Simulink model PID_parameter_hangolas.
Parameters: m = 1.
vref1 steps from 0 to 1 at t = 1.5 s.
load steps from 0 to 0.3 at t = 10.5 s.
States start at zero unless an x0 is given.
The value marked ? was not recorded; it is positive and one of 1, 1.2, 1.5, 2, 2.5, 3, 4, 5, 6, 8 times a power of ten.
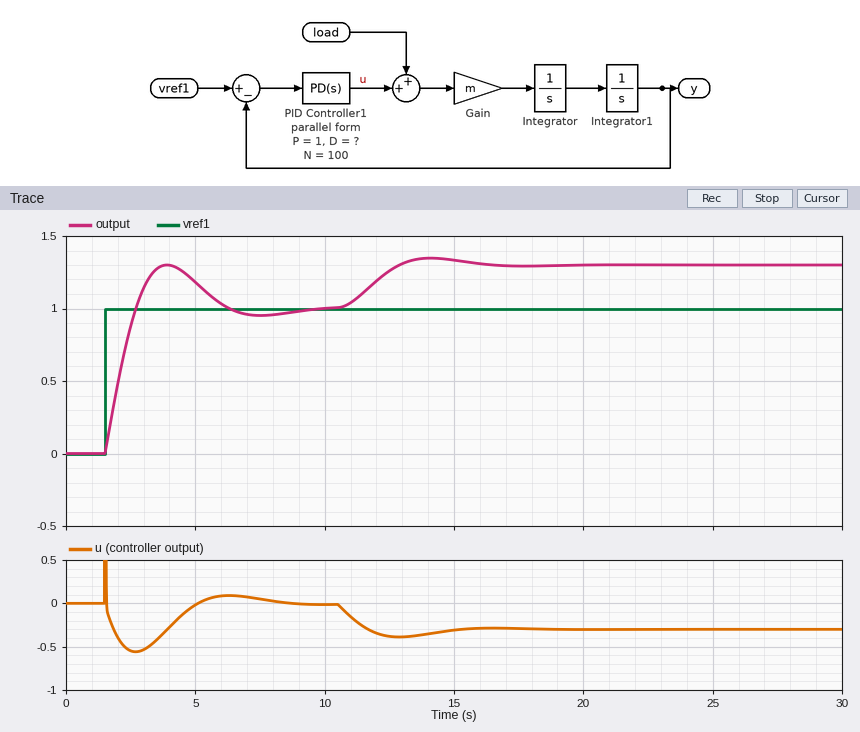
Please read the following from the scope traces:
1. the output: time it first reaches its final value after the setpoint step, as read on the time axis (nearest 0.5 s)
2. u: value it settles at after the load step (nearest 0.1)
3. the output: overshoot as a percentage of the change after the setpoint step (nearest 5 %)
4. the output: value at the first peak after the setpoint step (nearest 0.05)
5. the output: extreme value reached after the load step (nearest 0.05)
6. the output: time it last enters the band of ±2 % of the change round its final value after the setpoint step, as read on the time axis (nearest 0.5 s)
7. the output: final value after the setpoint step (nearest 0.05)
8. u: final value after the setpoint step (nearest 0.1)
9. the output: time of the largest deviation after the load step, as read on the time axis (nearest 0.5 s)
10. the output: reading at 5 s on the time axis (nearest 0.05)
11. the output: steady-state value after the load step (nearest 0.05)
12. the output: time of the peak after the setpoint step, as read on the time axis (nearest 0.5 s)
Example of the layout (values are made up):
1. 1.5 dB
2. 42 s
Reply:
1. 2.5 s
2. -0.3
3. 30 %
4. 1.30
5. 1.35
6. 9.0 s
7. 1.00
8. 0.0
9. 14.0 s
10. 1.20
11. 1.30
12. 4.0 s
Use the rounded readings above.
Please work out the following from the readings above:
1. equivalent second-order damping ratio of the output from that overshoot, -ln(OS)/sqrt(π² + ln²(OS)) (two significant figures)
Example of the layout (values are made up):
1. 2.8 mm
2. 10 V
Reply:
1. 0.36
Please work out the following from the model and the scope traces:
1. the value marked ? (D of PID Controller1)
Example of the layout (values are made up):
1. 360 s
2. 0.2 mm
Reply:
1. 1
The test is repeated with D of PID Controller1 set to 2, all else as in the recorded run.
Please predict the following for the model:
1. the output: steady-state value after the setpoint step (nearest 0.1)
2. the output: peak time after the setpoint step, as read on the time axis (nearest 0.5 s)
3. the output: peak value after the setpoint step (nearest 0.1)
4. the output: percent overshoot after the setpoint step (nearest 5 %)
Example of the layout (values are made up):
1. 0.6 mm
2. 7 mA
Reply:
1. 1.0
2. 3.5 s
3. 1.1
4. 15 %
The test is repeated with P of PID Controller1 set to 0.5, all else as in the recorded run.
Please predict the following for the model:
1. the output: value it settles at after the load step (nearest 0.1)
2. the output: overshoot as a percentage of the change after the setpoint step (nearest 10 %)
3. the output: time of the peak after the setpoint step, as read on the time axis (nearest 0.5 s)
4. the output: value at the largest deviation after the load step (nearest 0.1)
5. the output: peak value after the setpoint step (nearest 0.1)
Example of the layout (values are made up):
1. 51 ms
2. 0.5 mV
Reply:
1. 1.6
2. 20 %
3. 4.5 s
4. 1.6
5. 1.2
